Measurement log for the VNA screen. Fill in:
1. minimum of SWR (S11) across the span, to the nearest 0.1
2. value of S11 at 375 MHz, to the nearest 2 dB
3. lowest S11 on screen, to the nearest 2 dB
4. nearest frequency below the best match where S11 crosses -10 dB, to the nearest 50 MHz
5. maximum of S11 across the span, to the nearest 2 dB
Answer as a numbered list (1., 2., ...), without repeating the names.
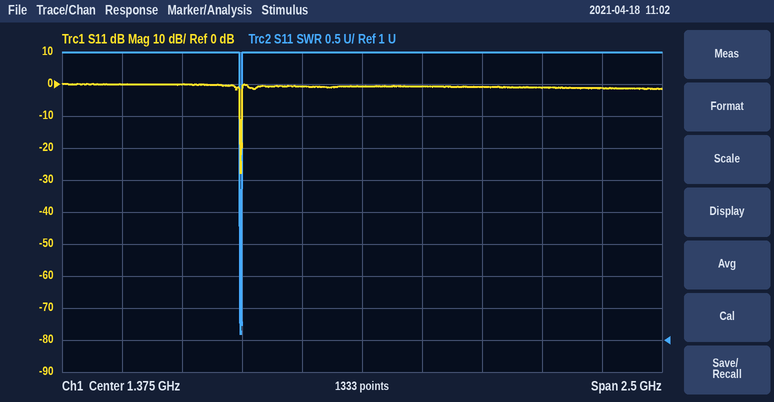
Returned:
1. 1.1
2. 0 dB
3. -28 dB
4. 850 MHz
5. 0 dB
